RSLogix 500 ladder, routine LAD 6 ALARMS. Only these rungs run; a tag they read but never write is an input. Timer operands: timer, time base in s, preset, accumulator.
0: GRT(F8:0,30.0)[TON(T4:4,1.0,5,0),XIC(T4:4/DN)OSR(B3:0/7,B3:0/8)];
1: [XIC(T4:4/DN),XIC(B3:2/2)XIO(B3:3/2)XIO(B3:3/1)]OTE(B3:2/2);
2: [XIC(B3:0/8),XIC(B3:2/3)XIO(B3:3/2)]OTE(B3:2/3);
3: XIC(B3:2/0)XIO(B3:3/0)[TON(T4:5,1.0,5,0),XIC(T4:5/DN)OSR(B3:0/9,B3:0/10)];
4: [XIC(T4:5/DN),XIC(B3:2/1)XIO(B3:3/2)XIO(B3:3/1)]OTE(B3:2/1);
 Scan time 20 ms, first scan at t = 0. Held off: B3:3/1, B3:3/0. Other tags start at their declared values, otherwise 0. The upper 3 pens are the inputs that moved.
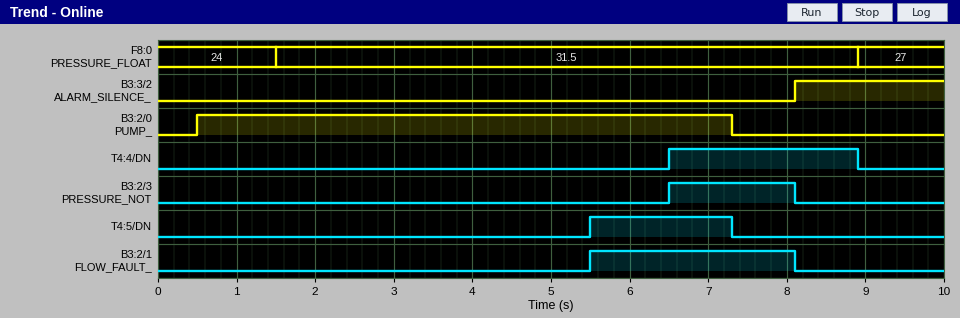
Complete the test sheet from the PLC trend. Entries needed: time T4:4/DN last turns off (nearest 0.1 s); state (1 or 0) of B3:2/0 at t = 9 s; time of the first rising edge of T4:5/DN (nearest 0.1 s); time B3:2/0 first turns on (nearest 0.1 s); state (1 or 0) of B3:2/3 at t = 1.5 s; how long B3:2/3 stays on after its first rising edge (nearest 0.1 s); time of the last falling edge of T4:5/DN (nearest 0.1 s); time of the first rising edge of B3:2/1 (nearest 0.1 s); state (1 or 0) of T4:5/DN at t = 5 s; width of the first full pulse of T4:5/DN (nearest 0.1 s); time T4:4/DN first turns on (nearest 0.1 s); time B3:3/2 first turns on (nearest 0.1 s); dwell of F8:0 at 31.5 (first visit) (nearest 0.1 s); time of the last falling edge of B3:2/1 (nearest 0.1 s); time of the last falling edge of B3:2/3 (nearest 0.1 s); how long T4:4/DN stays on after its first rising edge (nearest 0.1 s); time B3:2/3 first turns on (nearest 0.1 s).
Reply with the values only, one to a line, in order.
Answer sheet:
8.9 s
0
5.5 s
0.5 s
0
1.6 s
7.3 s
5.5 s
0
1.8 s
6.5 s
8.1 s
7.4 s
8.1 s
8.1 s
2.4 s
6.5 s
